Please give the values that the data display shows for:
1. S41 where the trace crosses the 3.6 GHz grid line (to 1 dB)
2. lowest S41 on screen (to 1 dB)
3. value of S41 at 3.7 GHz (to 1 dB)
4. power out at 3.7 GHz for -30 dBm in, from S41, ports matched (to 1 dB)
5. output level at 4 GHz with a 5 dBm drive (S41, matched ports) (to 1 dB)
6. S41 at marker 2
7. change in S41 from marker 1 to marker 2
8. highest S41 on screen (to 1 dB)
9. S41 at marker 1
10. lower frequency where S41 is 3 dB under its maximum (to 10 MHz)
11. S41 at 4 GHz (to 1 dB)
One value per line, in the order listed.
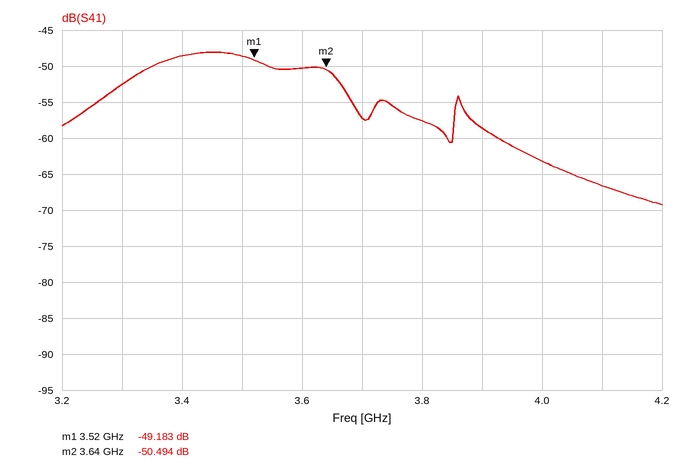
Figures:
-50 dB
-69 dB
-57 dB
-87 dBm
-58 dBm
-50.494 dB
-1.311 dB
-48 dB
-49.183 dB
3.33 GHz
-63 dB
